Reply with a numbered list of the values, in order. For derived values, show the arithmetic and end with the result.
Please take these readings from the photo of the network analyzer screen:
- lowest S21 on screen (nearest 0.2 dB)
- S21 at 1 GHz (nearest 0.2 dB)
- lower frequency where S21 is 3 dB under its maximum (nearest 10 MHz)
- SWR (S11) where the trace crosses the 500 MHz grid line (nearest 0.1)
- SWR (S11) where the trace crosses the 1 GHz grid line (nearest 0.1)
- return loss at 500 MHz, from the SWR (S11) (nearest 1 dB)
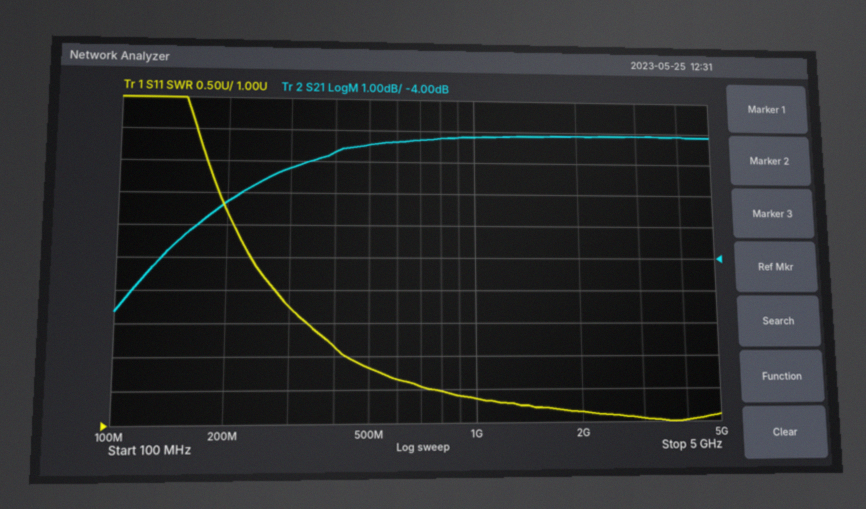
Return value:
1. -5.6 dB
2. -0.2 dB
3. 160 MHz
4. 1.8
5. 1.4
6. −20 log10((1.8 − 1)/(1.8 + 1)) ≈ 11 dB
